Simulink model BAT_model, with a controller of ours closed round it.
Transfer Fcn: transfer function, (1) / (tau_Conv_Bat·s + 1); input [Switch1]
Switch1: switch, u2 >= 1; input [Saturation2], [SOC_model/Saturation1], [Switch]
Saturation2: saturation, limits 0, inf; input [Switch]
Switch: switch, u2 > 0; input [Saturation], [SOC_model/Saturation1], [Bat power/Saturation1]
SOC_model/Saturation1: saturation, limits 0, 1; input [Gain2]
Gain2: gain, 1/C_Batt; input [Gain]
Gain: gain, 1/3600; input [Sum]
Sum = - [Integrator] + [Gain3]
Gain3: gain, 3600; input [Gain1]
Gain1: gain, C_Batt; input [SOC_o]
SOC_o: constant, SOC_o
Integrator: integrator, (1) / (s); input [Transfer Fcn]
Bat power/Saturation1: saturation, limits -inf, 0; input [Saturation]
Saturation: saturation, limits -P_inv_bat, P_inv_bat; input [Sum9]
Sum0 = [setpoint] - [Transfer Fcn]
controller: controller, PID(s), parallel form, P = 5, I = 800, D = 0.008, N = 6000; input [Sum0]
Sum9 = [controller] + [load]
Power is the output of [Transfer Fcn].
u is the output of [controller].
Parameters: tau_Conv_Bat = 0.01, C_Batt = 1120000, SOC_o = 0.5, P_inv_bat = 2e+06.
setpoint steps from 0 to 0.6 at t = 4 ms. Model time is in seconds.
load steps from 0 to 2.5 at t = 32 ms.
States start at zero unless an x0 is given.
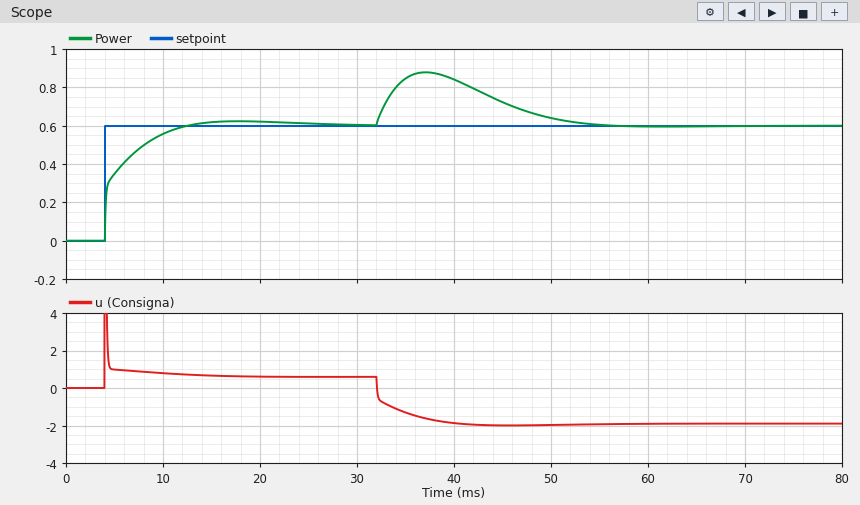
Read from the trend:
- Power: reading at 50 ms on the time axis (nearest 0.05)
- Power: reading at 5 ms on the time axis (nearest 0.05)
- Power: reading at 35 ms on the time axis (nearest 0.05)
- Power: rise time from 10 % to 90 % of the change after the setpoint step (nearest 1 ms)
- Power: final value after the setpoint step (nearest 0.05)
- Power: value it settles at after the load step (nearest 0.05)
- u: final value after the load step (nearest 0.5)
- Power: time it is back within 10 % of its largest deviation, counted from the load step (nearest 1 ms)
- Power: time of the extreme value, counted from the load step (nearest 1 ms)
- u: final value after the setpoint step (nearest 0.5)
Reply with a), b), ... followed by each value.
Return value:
a) 0.65
b) 0.35
c) 0.85
d) 5 ms
e) 0.60
f) 0.60
g) -2.0
h) 19 ms
i) 5 ms
j) 0.5
